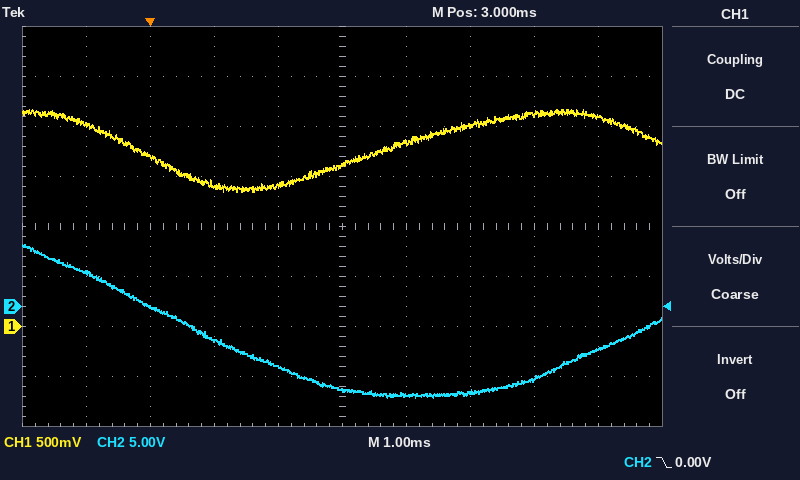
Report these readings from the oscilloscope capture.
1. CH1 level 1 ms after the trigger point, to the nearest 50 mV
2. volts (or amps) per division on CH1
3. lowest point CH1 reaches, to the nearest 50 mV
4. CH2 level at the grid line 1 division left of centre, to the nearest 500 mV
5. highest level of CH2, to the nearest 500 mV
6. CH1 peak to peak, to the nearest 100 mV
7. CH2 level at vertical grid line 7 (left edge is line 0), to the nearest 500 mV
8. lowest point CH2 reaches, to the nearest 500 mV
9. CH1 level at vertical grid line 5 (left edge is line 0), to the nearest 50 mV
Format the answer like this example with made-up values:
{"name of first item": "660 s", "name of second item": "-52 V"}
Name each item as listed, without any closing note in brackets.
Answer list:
{"CH1 level 1 ms after the trigger point, to the nearest 50 mV": "1.40 V", "volts (or amps) per division on CH1": "500 mV", "lowest point CH1 reaches, to the nearest 50 mV": "1.35 V", "CH2 level at the grid line 1 division left of centre, to the nearest 500 mV": "-6.0 V", "highest level of CH2, to the nearest 500 mV": "6.0 V", "CH1 peak to peak, to the nearest 100 mV": "800 mV", "CH2 level at vertical grid line 7 (left edge is line 0), to the nearest 500 mV": "-8.5 V", "lowest point CH2 reaches, to the nearest 500 mV": "-9.0 V", "CH1 level at vertical grid line 5 (left edge is line 0), to the nearest 50 mV": "1.60 V"}
